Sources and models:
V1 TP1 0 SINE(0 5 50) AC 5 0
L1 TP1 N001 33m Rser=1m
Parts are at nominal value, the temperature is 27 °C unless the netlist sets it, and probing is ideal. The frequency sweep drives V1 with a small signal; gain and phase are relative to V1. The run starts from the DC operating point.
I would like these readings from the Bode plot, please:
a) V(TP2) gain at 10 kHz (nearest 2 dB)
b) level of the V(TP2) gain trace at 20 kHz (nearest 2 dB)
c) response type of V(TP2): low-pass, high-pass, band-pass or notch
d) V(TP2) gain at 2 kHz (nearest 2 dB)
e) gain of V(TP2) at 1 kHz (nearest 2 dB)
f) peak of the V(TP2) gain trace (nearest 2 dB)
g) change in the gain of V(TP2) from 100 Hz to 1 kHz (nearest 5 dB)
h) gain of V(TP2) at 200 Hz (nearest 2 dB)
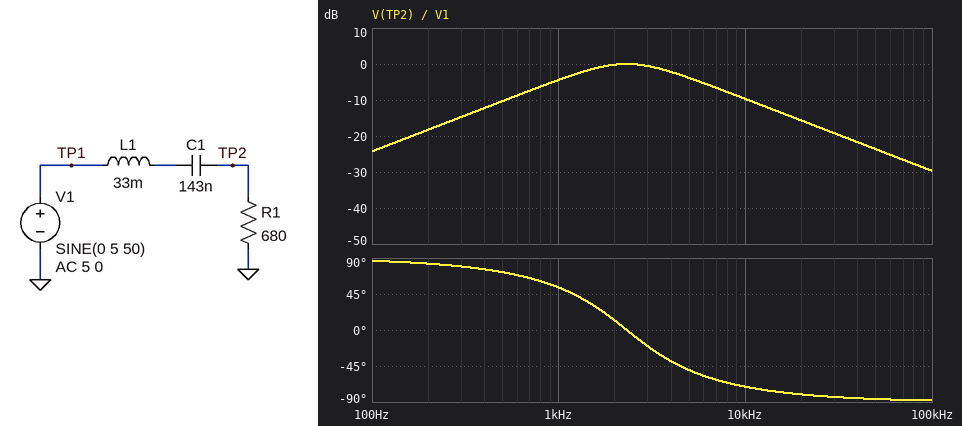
-10 dB
-16 dB
band-pass
0 dB
-4 dB
0 dB
20 dB
-18 dB
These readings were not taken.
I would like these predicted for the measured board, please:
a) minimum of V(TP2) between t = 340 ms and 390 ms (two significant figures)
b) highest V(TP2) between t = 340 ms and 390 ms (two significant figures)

-150 mV
150 mV
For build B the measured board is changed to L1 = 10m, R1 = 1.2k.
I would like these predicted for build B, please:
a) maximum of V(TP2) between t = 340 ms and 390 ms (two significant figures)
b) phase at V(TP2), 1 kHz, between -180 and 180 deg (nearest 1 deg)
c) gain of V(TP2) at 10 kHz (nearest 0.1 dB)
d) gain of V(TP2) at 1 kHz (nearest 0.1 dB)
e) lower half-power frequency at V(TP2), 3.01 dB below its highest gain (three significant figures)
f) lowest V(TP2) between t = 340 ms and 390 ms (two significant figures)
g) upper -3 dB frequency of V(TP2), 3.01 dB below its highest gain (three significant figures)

270 mV
41 deg
-0.7 dB
-2.5 dB
886 Hz
-270 mV
20.0 kHz
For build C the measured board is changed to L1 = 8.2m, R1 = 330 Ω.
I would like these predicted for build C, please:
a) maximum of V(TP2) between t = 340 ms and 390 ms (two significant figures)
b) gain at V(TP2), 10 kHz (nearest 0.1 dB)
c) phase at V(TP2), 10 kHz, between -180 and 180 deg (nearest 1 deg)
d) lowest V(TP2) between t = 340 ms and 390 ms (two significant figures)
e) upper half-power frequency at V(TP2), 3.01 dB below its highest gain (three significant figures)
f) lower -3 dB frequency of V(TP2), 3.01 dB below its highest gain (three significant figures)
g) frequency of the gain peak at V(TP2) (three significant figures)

74 mV
-4.0 dB
-51 deg
-74 mV
8.85 kHz
2.44 kHz
4.65 kHz
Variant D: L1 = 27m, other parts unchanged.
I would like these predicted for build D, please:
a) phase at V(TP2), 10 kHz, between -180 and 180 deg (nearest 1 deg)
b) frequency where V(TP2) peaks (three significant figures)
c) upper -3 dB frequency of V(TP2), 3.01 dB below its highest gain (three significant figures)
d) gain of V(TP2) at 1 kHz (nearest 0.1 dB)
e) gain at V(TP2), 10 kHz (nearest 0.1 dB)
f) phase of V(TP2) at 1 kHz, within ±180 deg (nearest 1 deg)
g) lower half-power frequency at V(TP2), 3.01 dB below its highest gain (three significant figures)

-67 deg
2.56 kHz
5.26 kHz
-4.7 dB
-8.1 dB
54 deg
1.25 kHz
